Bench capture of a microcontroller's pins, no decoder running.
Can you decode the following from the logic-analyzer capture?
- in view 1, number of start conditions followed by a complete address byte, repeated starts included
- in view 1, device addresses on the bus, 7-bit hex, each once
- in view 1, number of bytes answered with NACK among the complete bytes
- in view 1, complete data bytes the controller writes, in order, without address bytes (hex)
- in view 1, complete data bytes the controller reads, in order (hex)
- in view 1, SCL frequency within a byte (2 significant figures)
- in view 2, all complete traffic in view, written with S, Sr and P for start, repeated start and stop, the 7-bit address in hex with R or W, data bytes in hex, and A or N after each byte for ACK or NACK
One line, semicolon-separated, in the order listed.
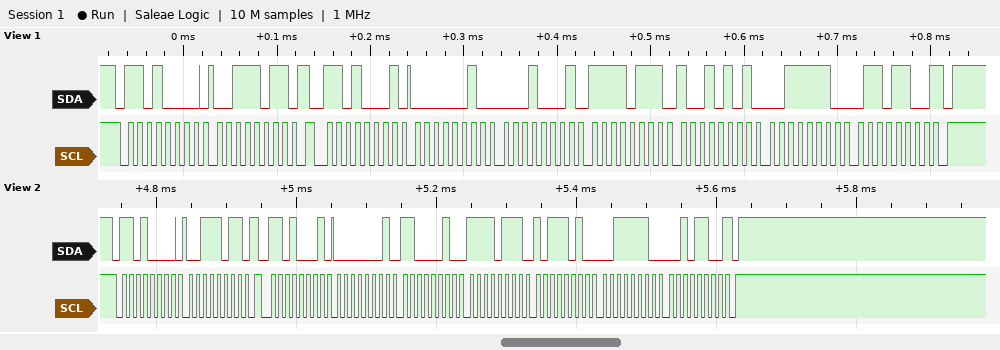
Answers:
2; 0x68; 1; 3B; 02 11 F7 95 3E 6C; 100 kHz; S 68W A 3B A Sr 68R A 01 A C2 A F7 A BA A 3E A 2C N P
